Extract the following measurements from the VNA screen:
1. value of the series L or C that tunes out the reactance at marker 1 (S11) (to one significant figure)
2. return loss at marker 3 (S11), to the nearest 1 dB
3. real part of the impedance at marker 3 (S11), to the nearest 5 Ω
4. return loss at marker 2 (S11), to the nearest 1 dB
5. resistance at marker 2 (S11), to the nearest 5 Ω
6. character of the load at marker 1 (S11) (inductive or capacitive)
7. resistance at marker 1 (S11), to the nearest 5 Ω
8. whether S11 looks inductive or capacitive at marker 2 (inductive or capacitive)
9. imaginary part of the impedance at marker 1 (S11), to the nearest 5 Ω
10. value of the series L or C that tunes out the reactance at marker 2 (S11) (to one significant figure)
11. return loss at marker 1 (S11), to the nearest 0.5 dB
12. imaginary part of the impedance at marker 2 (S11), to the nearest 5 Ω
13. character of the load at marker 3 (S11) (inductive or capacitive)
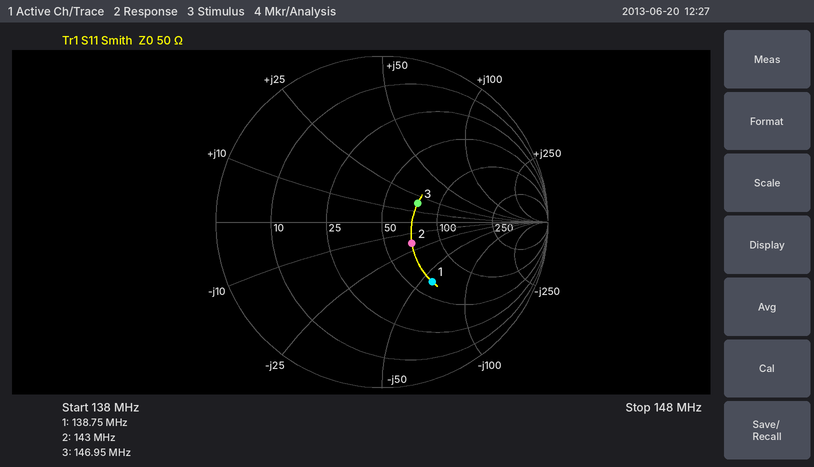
70 nH
12 dB
75 Ω
13 dB
70 Ω
capacitive
65 Ω
capacitive
-60 Ω
20 nH
6.5 dB
-20 Ω
inductive
